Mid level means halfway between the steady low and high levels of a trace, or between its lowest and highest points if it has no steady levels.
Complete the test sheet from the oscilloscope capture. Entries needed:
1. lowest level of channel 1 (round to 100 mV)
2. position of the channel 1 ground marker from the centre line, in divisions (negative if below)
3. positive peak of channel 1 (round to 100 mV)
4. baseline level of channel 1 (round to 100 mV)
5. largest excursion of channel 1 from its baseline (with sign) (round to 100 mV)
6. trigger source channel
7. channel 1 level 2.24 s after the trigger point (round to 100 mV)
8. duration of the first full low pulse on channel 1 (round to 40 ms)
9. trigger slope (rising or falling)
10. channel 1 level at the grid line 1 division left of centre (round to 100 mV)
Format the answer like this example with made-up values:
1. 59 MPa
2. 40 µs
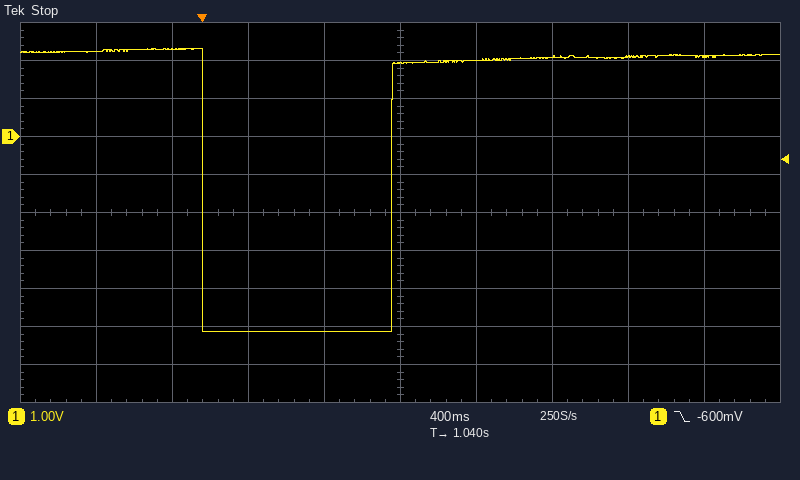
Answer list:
1. -5.1 V
2. +2.0 div
3. 2.3 V
4. 2.1 V
5. -7.2 V
6. channel 1
7. 2.1 V
8. 1.00 s
9. falling
10. -5.1 V
